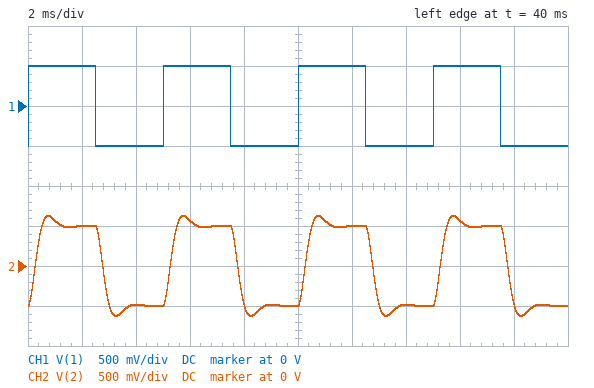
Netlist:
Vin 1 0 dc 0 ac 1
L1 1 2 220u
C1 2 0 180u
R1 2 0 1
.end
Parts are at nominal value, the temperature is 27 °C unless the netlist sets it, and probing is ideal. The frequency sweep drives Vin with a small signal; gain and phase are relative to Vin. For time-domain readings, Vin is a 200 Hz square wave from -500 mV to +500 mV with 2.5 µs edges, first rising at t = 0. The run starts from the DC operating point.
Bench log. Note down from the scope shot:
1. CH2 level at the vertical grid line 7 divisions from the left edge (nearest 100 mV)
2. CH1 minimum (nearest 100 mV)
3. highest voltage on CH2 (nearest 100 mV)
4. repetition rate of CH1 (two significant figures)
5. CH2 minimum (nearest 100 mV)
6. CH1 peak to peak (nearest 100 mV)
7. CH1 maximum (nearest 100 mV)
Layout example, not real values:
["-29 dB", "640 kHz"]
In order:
["-500 mV", "-500 mV", "600 mV", "200 Hz", "-600 mV", "1.0 V", "500 mV"]
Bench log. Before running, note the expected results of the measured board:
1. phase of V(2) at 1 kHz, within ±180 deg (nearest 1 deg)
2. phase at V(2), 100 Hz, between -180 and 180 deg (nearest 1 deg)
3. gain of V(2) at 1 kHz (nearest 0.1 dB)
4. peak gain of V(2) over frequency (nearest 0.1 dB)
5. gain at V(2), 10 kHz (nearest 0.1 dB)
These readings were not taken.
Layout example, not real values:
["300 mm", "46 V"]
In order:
["-112 deg", "-8 deg", "-3.5 dB", "0.7 dB", "-43.9 dB"]
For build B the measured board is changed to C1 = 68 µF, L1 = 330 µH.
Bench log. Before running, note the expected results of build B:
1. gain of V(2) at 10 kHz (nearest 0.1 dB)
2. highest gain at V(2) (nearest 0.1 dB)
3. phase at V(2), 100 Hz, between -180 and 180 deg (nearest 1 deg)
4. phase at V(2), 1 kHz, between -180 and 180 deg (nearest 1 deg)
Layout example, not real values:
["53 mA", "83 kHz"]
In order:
["-39.1 dB", "0 dB", "-12 deg", "-87 deg"]
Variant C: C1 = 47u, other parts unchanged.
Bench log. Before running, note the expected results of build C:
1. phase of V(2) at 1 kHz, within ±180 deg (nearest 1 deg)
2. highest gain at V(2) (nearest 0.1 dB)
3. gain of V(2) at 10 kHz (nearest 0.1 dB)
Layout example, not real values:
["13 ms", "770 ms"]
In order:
["-67 deg", "0 dB", "-32.5 dB"]
